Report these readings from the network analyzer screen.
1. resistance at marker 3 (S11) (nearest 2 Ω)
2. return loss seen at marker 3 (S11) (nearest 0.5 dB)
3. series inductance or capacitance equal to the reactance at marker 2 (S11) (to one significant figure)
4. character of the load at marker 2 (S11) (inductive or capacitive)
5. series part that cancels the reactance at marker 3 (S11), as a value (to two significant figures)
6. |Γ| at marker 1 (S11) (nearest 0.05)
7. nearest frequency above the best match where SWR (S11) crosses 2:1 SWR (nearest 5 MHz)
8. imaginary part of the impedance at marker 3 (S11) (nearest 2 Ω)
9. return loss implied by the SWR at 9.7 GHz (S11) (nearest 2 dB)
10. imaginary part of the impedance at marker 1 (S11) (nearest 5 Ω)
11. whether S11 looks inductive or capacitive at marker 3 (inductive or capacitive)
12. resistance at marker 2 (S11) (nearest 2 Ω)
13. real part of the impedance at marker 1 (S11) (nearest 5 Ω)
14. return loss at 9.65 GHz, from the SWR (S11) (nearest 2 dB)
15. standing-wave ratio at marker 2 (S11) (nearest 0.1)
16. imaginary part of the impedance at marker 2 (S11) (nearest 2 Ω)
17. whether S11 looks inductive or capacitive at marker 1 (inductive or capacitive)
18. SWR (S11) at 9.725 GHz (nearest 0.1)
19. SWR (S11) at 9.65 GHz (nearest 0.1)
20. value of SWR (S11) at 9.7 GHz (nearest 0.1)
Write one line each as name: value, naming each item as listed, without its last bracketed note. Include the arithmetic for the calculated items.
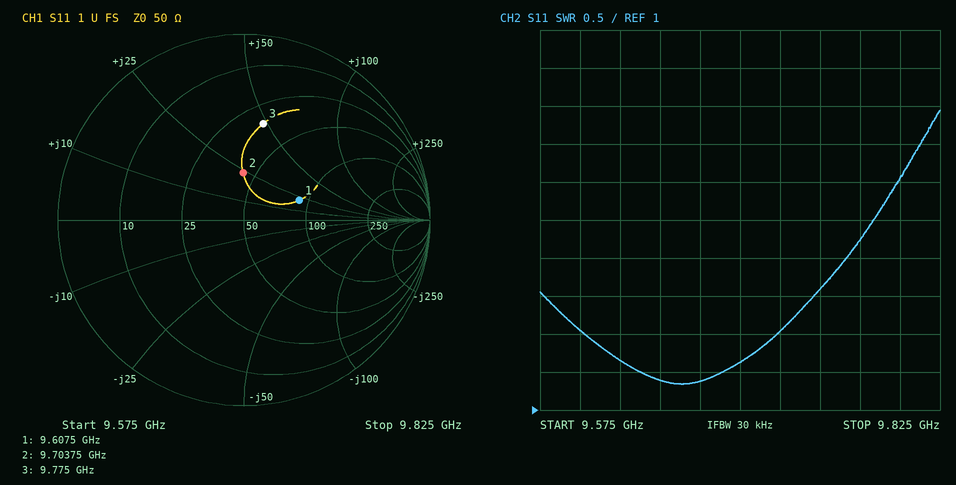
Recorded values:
resistance at marker 3 (S11): 34 Ω
return loss seen at marker 3 (S11): 5.5 dB
series inductance or capacitance equal to the reactance at marker 2 (S11): L = 24 Ω/(2π × 9.70375 GHz) ≈ 394 pH, so 400 pH to one significant figure
character of the load at marker 2 (S11): inductive
series part that cancels the reactance at marker 3 (S11), as a value: C = 1/(2π × 9.775 GHz × 48 Ω) ≈ 339 fF, so 340 fF to two significant figures
|Γ| at marker 1 (S11): 0.30
nearest frequency above the best match where SWR (S11) crosses 2:1 SWR: 9.725 GHz
imaginary part of the impedance at marker 3 (S11): +48 Ω
return loss implied by the SWR at 9.7 GHz (S11): −20 log10((1.6 − 1)/(1.6 + 1)) ≈ 12.7 dB, so 12 dB to the nearest 2 dB
imaginary part of the impedance at marker 1 (S11): +20 Ω
whether S11 looks inductive or capacitive at marker 3: inductive
resistance at marker 2 (S11): 44 Ω
real part of the impedance at marker 1 (S11): 90 Ω
return loss at 9.65 GHz, from the SWR (S11): −20 log10((1.4 − 1)/(1.4 + 1)) ≈ 16 dB
standing-wave ratio at marker 2 (S11): 1.7
imaginary part of the impedance at marker 2 (S11): +24 Ω
whether S11 looks inductive or capacitive at marker 1: inductive
SWR (S11) at 9.725 GHz: 2.0
SWR (S11) at 9.65 GHz: 1.4
value of SWR (S11) at 9.7 GHz: 1.6
